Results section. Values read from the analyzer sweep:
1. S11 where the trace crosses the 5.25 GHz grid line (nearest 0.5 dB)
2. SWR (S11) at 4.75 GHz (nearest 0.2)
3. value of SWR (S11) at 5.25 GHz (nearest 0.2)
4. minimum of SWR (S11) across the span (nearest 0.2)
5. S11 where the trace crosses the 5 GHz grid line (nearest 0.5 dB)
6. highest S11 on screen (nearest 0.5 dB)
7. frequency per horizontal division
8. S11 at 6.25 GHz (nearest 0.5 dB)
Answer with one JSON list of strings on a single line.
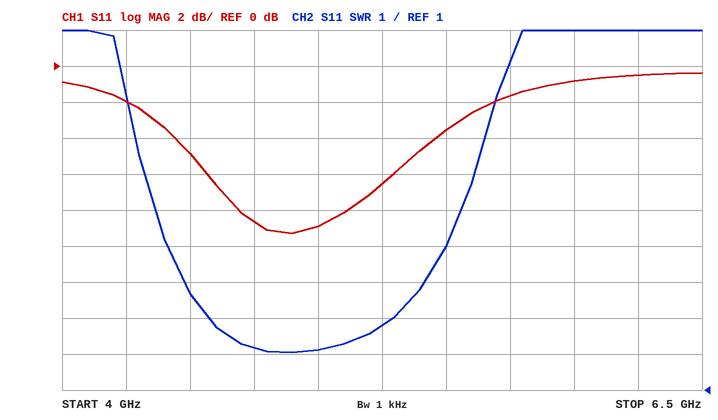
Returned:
["-6.5 dB", "2.2", "2.8", "2.0", "-9.0 dB", "-0.5 dB", "250 MHz", "-0.5 dB"]
